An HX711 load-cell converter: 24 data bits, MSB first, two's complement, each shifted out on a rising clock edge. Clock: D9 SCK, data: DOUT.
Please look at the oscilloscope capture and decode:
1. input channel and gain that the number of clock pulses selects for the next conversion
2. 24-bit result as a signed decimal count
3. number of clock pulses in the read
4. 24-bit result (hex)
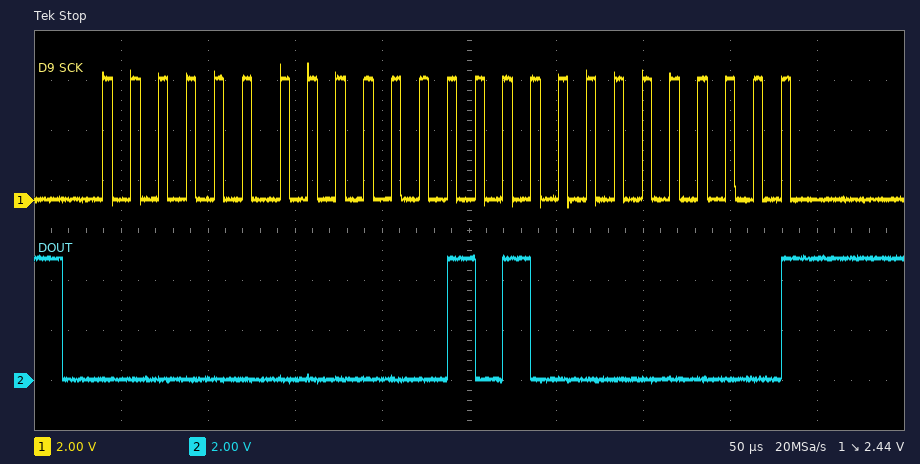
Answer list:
channel A, gain 128
2560
25
0x000A00
